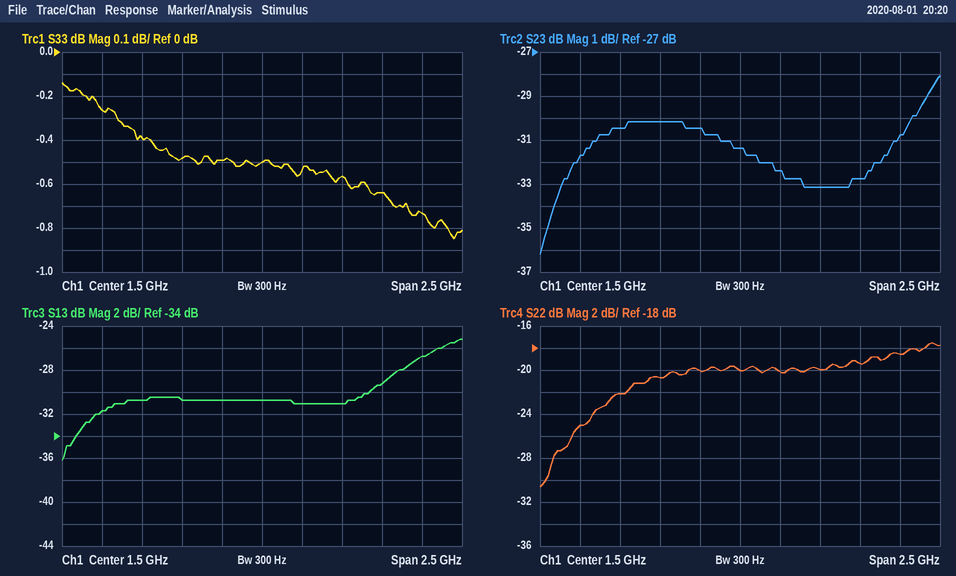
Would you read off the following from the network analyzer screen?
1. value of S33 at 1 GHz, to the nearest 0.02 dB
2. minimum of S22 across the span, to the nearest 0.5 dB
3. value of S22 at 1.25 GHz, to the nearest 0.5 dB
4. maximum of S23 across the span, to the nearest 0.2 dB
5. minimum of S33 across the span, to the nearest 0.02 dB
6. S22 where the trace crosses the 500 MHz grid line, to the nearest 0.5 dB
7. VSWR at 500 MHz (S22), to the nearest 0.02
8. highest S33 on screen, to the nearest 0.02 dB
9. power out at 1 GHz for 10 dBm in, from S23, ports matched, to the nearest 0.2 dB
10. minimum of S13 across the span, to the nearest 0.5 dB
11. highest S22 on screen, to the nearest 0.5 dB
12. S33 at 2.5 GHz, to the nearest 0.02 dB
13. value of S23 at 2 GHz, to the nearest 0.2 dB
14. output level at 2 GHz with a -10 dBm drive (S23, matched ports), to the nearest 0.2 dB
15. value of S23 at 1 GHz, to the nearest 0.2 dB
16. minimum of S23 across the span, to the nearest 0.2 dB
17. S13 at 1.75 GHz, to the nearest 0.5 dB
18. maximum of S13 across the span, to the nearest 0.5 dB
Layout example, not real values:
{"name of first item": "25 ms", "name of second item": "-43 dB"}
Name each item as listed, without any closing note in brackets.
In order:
{"value of S33 at 1 GHz, to the nearest 0.02 dB": "-0.48 dB", "minimum of S22 across the span, to the nearest 0.5 dB": "-30.5 dB", "value of S22 at 1.25 GHz, to the nearest 0.5 dB": "-20.0 dB", "maximum of S23 across the span, to the nearest 0.2 dB": "-28.0 dB", "minimum of S33 across the span, to the nearest 0.02 dB": "-0.84 dB", "S22 where the trace crosses the 500 MHz grid line, to the nearest 0.5 dB": "-25.0 dB", "VSWR at 500 MHz (S22), to the nearest 0.02": "1.12", "highest S33 on screen, to the nearest 0.02 dB": "-0.14 dB", "power out at 1 GHz for 10 dBm in, from S23, ports matched, to the nearest 0.2 dB": "-20.2 dBm", "minimum of S13 across the span, to the nearest 0.5 dB": "-36.0 dB", "highest S22 on screen, to the nearest 0.5 dB": "-17.5 dB", "S33 at 2.5 GHz, to the nearest 0.02 dB": "-0.74 dB", "value of S23 at 2 GHz, to the nearest 0.2 dB": "-33.2 dB", "output level at 2 GHz with a -10 dBm drive (S23, matched ports), to the nearest 0.2 dB": "-43.2 dBm", "value of S23 at 1 GHz, to the nearest 0.2 dB": "-30.2 dB", "minimum of S23 across the span, to the nearest 0.2 dB": "-36.2 dB", "S13 at 1.75 GHz, to the nearest 0.5 dB": "-31.0 dB", "maximum of S13 across the span, to the nearest 0.5 dB": "-25.0 dB"}
